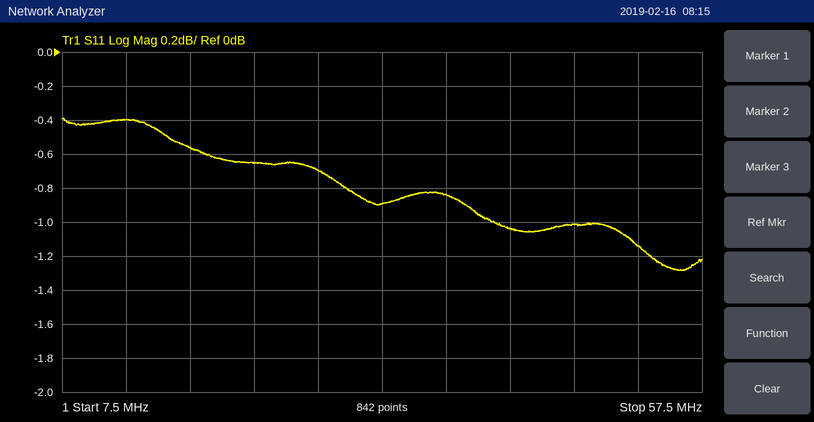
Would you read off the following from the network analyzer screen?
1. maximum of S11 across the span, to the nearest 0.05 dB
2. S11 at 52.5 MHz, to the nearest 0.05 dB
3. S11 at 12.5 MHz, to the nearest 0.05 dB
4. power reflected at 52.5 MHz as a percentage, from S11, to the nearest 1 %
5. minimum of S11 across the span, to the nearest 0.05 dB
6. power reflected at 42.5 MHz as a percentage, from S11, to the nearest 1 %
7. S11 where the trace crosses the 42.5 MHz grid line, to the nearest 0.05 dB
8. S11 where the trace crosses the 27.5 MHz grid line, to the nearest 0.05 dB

-0.40 dB
-1.15 dB
-0.40 dB
77 %
-1.30 dB
79 %
-1.05 dB
-0.70 dB
